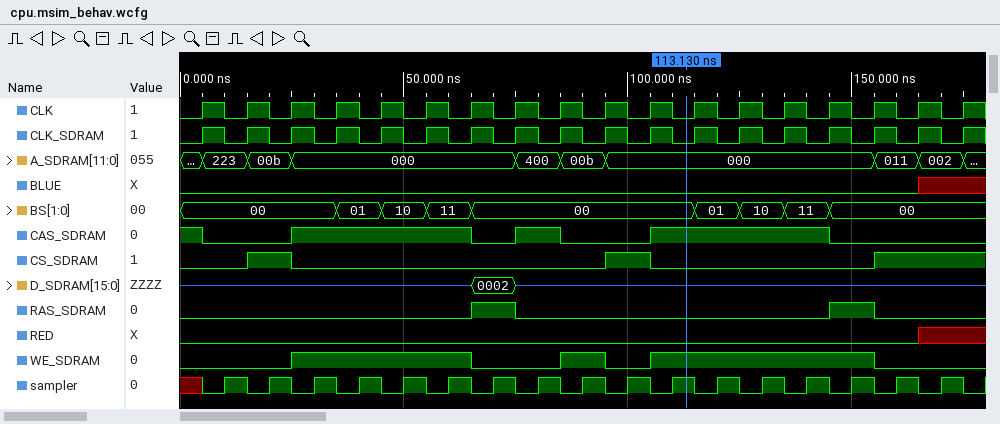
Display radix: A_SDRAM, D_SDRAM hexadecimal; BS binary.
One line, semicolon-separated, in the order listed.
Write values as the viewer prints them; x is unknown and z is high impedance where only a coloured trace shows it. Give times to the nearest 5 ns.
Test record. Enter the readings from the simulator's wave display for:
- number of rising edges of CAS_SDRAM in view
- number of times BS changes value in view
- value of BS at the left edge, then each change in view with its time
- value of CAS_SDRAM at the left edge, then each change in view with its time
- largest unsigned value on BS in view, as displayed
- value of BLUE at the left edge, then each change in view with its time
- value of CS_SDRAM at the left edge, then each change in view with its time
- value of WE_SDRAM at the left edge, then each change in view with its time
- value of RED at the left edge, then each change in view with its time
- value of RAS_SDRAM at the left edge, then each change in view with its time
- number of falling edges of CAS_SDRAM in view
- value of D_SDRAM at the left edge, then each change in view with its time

3; 8; 00, 01 at 35 ns, 10 at 45 ns, 11 at 55 ns, 00 at 65 ns, 01 at 115 ns, 10 at 125 ns, 11 at 135 ns, 00 at 145 ns; 1, 0 at 5 ns, 1 at 25 ns, 0 at 65 ns, 1 at 75 ns, 0 at 85 ns, 1 at 105 ns, 0 at 145 ns; 11; 0, x at 165 ns; 0, 1 at 15 ns, 0 at 25 ns, 1 at 95 ns, 0 at 105 ns, 1 at 155 ns; 0, 1 at 25 ns, 0 at 65 ns, 1 at 85 ns, 0 at 95 ns, 1 at 105 ns, 0 at 155 ns; 0, x at 165 ns; 0, 1 at 65 ns, 0 at 75 ns, 1 at 145 ns, 0 at 155 ns; 4; z, 0002 at 65 ns, z at 75 ns
